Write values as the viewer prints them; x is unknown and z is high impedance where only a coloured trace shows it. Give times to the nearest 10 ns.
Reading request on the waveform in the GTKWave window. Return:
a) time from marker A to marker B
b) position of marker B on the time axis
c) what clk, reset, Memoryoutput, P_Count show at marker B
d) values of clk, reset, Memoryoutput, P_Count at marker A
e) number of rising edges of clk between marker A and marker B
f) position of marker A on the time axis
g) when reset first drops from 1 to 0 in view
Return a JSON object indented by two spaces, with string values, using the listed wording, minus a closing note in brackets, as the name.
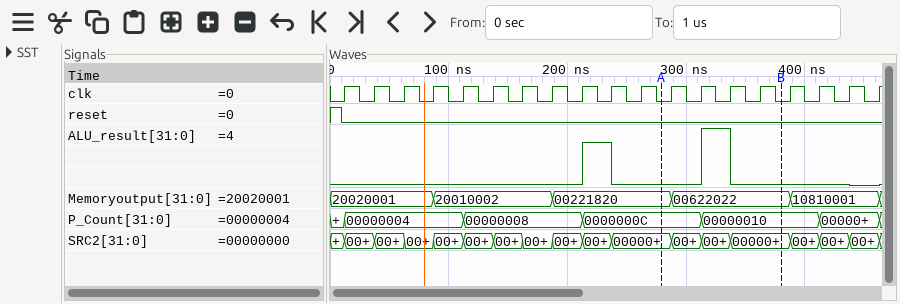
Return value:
{
  "time from marker A to marker B": "100 ns",
  "position of marker B on the time axis": "380 ns",
  "what clk, reset, Memoryoutput, P_Count show at marker B": "clk=0, reset=0, Memoryoutput=00622022, P_Count=00000010",
  "values of clk, reset, Memoryoutput, P_Count at marker A": "clk=0, reset=0, Memoryoutput=00221820, P_Count=0000000C",
  "number of rising edges of clk between marker A and marker B": "4",
  "position of marker A on the time axis": "280 ns",
  "when reset first drops from 1 to 0 in view": "10 ns"
}
